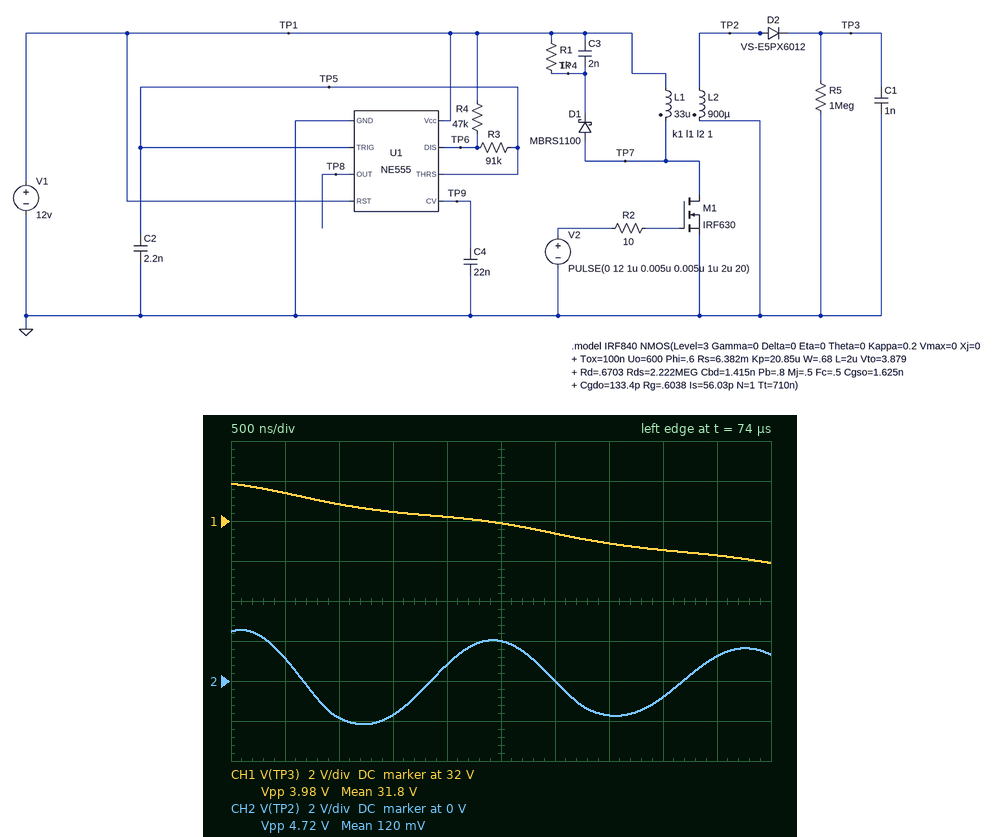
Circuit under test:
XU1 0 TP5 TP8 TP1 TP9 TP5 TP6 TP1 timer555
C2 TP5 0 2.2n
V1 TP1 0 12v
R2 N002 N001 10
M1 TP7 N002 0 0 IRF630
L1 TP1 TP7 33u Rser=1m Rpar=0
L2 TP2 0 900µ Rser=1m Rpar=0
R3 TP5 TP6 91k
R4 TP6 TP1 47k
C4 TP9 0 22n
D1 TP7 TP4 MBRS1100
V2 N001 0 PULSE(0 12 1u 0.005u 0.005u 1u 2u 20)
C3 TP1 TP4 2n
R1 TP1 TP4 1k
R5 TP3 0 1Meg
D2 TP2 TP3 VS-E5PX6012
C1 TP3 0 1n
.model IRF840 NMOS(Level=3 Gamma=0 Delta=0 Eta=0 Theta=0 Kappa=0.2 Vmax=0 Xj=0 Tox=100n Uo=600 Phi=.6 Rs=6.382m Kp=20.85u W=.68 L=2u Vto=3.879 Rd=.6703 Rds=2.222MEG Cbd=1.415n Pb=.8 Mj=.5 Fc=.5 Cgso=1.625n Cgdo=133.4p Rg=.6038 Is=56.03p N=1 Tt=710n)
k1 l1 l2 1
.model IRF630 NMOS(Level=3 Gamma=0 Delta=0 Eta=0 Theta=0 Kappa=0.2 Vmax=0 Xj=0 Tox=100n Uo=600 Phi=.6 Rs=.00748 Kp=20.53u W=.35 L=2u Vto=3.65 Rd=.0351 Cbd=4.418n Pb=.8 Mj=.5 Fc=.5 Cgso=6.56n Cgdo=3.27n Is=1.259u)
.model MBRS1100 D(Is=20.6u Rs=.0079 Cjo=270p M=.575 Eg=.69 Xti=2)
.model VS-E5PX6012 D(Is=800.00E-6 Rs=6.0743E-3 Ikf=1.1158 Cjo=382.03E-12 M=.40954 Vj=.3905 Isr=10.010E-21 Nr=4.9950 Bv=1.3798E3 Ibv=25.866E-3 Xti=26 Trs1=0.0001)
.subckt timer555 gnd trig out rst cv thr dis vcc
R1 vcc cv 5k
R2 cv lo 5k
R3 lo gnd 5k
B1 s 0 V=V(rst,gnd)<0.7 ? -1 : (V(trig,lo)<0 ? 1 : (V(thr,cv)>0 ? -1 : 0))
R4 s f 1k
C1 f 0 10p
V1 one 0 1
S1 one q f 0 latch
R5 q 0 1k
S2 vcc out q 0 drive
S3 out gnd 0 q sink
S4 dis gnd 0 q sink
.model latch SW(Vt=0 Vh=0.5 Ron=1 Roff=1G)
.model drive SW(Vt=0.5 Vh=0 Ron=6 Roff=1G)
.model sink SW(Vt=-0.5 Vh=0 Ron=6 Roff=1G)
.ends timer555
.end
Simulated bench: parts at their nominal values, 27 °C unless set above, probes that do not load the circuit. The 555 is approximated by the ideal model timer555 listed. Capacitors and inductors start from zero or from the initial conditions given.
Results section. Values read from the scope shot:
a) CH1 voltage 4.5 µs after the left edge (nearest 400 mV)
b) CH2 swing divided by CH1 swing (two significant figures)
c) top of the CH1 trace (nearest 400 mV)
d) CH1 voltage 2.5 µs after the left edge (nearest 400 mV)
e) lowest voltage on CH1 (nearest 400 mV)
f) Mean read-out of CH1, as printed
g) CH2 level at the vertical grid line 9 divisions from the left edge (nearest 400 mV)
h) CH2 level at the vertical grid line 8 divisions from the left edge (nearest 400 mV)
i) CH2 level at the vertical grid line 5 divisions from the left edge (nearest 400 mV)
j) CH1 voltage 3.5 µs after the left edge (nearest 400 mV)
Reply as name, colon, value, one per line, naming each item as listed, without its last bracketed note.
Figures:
CH1 voltage 4.5 µs after the left edge: 30.4 V
CH2 swing divided by CH1 swing: 1.2
top of the CH1 trace: 34.0 V
CH1 voltage 2.5 µs after the left edge: 32.0 V
lowest voltage on CH1: 30.0 V
Mean read-out of CH1, as printed: 31.8 V
CH2 level at the vertical grid line 9 divisions from the left edge: 1.2 V
CH2 level at the vertical grid line 8 divisions from the left edge: -800 mV
CH2 level at the vertical grid line 5 divisions from the left edge: 2.0 V
CH1 voltage 3.5 µs after the left edge: 30.8 V
